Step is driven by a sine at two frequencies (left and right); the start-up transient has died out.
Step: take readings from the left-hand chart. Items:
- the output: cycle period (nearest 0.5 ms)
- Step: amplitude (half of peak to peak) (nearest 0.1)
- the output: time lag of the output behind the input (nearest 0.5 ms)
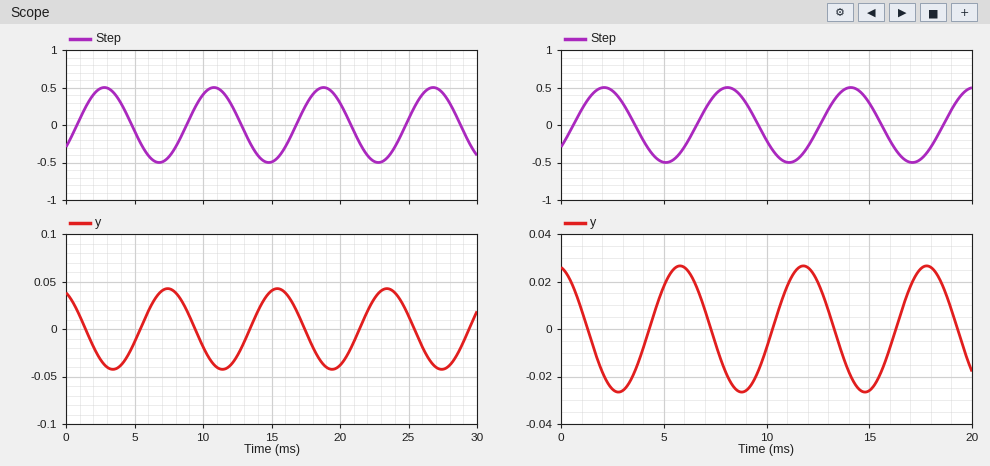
8.0 ms
0.5
4.5 ms
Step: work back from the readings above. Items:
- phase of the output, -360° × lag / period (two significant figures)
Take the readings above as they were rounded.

-200°
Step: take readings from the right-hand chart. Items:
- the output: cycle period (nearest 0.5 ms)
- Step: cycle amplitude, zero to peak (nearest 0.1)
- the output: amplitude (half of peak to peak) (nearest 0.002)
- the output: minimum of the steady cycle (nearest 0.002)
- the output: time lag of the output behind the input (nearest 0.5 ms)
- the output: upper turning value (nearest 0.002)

6.0 ms
0.5
0.026
-0.026
3.5 ms
0.026
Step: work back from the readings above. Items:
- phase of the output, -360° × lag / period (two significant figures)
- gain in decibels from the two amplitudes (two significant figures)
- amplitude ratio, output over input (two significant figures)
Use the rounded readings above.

-210°
-26 dB
0.052
